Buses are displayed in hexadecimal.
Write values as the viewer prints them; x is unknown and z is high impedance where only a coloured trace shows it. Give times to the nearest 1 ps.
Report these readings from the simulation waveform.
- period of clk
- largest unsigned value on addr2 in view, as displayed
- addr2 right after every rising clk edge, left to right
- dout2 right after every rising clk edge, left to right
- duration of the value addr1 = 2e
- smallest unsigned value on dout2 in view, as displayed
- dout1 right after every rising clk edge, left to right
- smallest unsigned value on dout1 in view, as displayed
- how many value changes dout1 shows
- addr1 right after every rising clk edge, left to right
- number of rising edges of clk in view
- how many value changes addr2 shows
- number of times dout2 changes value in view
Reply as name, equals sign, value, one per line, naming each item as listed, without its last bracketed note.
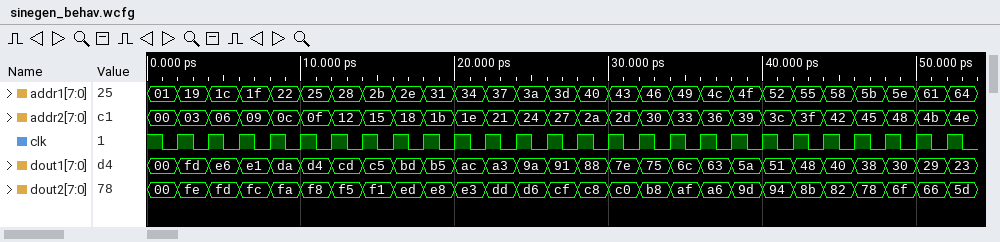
period of clk = 2 ps
largest unsigned value on addr2 in view, as displayed = 4e
addr2 right after every rising clk edge, left to right = 03, 06, 09, 0c, 0f, 12, 15, 18, 1b, 1e, 21, 24, 27, 2a, 2d, 30, 33, 36, 39, 3c, 3f, 42, 45, 48, 4b, 4e
dout2 right after every rising clk edge, left to right = fe, fd, fc, fa, f8, f5, f1, ed, e8, e3, dd, d6, cf, c8, c0, b8, af, a6, 9d, 94, 8b, 82, 78, 6f, 66, 5d
duration of the value addr1 = 2e = 2 ps
smallest unsigned value on dout2 in view, as displayed = 00
dout1 right after every rising clk edge, left to right = fd, e6, e1, da, d4, cd, c5, bd, b5, ac, a3, 9a, 91, 88, 7e, 75, 6c, 63, 5a, 51, 48, 40, 38, 30, 29, 23
smallest unsigned value on dout1 in view, as displayed = 00
how many value changes dout1 shows = 26
addr1 right after every rising clk edge, left to right = 19, 1c, 1f, 22, 25, 28, 2b, 2e, 31, 34, 37, 3a, 3d, 40, 43, 46, 49, 4c, 4f, 52, 55, 58, 5b, 5e, 61, 64
number of rising edges of clk in view = 26
how many value changes addr2 shows = 26
number of times dout2 changes value in view = 26
